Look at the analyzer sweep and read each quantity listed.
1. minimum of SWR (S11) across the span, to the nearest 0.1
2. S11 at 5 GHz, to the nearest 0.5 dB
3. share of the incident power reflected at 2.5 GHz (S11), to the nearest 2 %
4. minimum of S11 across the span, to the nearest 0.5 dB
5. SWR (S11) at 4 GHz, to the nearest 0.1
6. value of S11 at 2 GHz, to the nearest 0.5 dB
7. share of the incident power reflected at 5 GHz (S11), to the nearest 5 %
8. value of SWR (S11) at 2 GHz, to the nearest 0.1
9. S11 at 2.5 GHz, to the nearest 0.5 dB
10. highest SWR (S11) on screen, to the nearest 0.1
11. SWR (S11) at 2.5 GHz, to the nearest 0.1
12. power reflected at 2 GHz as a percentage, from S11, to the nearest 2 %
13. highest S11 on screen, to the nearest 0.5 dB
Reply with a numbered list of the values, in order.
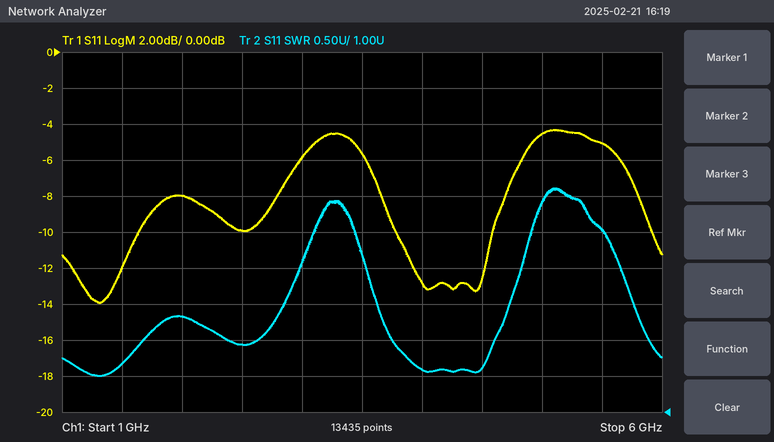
1. 1.5
2. -4.5 dB
3. 10 %
4. -14.0 dB
5. 1.6
6. -8.0 dB
7. 35 %
8. 2.3
9. -10.0 dB
10. 4.1
11. 1.9
12. 16 %
13. -4.5 dB
